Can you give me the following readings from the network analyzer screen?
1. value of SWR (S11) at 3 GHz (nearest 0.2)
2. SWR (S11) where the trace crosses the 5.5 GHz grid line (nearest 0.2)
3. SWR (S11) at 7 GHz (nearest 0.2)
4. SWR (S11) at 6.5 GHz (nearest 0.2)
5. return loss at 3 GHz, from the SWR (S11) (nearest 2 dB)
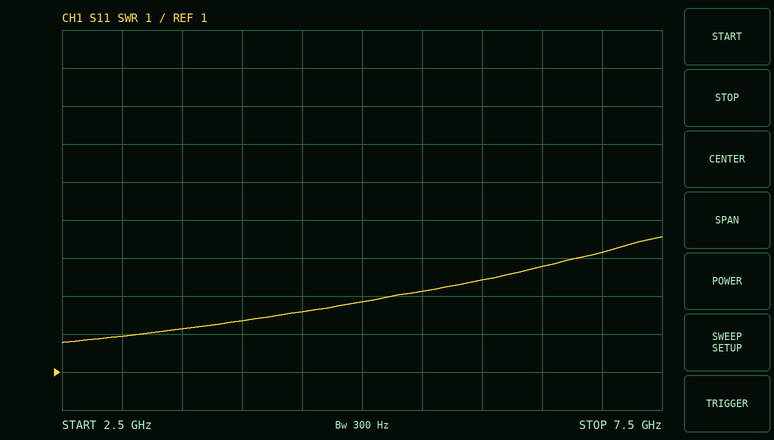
2.0
3.2
4.2
3.8
10 dB
